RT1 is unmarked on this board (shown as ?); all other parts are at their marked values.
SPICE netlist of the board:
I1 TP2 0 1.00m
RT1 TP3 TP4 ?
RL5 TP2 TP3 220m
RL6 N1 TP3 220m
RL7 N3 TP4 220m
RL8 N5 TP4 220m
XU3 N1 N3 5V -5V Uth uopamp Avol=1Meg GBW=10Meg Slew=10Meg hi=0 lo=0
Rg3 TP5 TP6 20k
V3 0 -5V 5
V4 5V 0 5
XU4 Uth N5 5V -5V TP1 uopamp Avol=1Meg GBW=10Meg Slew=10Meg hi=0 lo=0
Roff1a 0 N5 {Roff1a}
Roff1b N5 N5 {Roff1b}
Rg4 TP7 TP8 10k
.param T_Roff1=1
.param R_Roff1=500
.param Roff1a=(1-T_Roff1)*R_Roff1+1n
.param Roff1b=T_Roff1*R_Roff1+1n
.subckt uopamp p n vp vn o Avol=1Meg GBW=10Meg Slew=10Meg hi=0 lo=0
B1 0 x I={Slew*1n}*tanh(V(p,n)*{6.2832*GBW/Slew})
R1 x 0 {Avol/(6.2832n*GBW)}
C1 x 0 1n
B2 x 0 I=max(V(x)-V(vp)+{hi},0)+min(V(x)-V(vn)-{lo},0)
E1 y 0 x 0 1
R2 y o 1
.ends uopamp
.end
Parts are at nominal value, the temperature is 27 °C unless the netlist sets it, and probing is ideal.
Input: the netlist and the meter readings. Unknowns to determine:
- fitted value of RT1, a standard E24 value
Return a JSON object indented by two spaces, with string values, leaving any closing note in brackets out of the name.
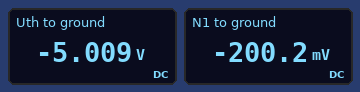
{
  "fitted value of RT1, a standard E24 value": "200 Ω"
}
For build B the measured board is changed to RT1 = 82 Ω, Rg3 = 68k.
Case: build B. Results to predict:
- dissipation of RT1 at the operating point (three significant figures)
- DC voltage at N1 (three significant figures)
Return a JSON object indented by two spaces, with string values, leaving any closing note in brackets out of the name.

{
  "dissipation of RT1 at the operating point": "82.0 µW",
  "DC voltage at N1": "-82.2 mV"
}
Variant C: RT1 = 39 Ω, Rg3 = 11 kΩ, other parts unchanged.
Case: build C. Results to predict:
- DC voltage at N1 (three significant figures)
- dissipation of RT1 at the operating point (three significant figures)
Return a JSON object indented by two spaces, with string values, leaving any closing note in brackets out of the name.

{
  "DC voltage at N1": "-39.2 mV",
  "dissipation of RT1 at the operating point": "39.0 µW"
}
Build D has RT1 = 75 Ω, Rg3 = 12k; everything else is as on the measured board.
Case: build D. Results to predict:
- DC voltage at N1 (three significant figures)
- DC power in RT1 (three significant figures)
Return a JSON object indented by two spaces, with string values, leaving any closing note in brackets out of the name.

{
  "DC voltage at N1": "-75.2 mV",
  "DC power in RT1": "75.0 µW"
}
